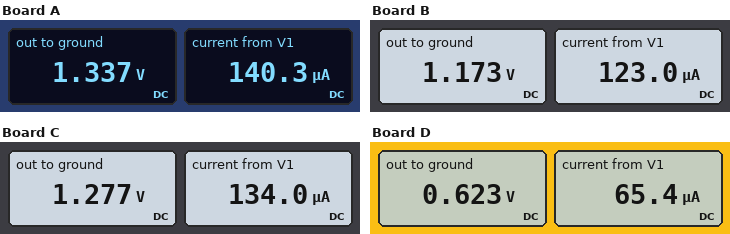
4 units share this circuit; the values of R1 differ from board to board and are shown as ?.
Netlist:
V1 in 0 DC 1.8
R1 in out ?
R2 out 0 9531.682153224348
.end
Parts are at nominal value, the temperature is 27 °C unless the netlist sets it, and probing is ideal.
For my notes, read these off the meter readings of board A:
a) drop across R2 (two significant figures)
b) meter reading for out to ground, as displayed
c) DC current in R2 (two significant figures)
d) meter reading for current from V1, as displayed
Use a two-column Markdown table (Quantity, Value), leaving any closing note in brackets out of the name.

| Quantity | Value |
|---|---|
| drop across R2 | 1.3 V |
| meter reading for out to ground, as displayed | 1.337 V |
| DC current in R2 | 140 µA |
| meter reading for current from V1, as displayed | 140.3 µA |
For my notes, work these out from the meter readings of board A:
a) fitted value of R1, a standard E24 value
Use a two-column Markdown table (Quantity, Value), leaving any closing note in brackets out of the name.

| Quantity | Value |
|---|---|
| fitted value of R1, a standard E24 value | 3.3 kΩ |
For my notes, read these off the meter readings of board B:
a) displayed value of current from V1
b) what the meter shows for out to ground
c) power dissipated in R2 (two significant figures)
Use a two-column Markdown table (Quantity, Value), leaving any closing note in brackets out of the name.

| Quantity | Value |
|---|---|
| displayed value of current from V1 | 123.0 µA |
| what the meter shows for out to ground | 1.173 V |
| power dissipated in R2 | 140 µW |
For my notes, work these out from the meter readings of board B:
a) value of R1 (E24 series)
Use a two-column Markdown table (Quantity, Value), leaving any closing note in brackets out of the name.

| Quantity | Value |
|---|---|
| value of R1 | 5.1 kΩ |
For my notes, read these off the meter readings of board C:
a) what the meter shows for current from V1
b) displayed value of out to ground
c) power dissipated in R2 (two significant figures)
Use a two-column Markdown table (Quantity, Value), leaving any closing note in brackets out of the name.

| Quantity | Value |
|---|---|
| what the meter shows for current from V1 | 134.0 µA |
| displayed value of out to ground | 1.277 V |
| power dissipated in R2 | 170 µW |
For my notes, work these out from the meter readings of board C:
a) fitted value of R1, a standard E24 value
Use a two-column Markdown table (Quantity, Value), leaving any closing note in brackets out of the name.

| Quantity | Value |
|---|---|
| fitted value of R1, a standard E24 value | 3.9 kΩ |
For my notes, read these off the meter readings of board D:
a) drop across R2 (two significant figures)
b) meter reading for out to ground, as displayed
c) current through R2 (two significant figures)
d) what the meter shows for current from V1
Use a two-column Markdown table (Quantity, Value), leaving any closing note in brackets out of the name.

| Quantity | Value |
|---|---|
| drop across R2 | 620 mV |
| meter reading for out to ground, as displayed | 0.623 V |
| current through R2 | 65 µA |
| what the meter shows for current from V1 | 65.4 µA |
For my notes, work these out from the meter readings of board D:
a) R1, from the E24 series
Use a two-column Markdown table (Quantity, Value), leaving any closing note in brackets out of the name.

| Quantity | Value |
|---|---|
| R1, from the E24 series | 18 kΩ |
